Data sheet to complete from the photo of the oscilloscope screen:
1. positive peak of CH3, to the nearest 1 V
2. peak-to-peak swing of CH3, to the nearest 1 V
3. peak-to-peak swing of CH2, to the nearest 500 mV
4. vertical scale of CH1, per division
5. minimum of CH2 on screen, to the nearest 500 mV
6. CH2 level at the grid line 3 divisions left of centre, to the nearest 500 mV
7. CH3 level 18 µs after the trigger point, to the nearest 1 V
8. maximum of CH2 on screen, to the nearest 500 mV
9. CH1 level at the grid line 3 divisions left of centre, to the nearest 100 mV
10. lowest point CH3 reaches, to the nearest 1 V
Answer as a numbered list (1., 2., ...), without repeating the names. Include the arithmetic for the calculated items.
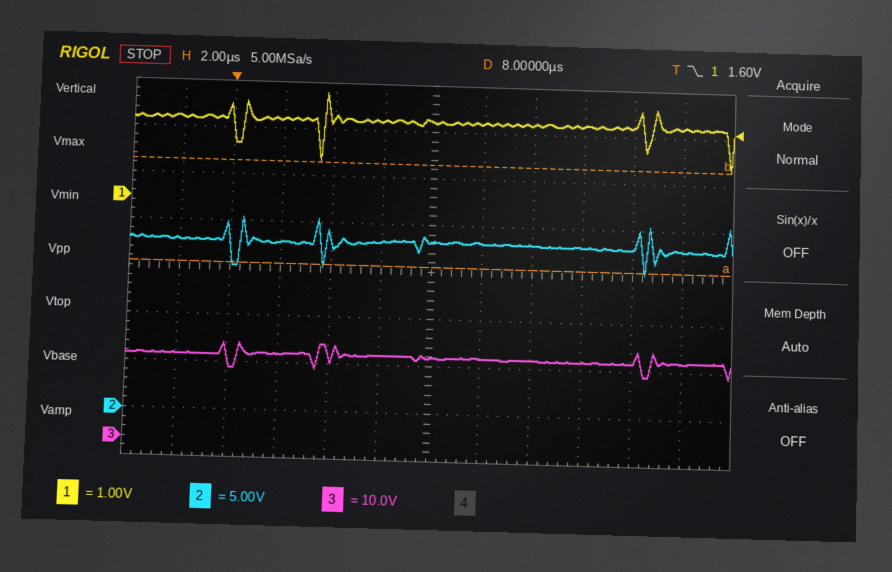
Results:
1. 20 V
2. 20 V − (15 V) = 5 V
3. 20.5 V − (15.5 V) = 5.0 V
4. 1 V
5. 15.5 V
6. 18.0 V
7. 18 V
8. 20.5 V
9. 1.7 V
10. 15 V
